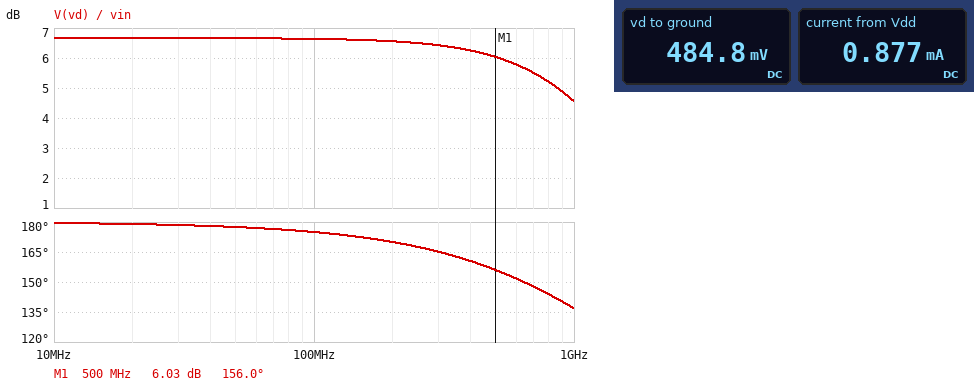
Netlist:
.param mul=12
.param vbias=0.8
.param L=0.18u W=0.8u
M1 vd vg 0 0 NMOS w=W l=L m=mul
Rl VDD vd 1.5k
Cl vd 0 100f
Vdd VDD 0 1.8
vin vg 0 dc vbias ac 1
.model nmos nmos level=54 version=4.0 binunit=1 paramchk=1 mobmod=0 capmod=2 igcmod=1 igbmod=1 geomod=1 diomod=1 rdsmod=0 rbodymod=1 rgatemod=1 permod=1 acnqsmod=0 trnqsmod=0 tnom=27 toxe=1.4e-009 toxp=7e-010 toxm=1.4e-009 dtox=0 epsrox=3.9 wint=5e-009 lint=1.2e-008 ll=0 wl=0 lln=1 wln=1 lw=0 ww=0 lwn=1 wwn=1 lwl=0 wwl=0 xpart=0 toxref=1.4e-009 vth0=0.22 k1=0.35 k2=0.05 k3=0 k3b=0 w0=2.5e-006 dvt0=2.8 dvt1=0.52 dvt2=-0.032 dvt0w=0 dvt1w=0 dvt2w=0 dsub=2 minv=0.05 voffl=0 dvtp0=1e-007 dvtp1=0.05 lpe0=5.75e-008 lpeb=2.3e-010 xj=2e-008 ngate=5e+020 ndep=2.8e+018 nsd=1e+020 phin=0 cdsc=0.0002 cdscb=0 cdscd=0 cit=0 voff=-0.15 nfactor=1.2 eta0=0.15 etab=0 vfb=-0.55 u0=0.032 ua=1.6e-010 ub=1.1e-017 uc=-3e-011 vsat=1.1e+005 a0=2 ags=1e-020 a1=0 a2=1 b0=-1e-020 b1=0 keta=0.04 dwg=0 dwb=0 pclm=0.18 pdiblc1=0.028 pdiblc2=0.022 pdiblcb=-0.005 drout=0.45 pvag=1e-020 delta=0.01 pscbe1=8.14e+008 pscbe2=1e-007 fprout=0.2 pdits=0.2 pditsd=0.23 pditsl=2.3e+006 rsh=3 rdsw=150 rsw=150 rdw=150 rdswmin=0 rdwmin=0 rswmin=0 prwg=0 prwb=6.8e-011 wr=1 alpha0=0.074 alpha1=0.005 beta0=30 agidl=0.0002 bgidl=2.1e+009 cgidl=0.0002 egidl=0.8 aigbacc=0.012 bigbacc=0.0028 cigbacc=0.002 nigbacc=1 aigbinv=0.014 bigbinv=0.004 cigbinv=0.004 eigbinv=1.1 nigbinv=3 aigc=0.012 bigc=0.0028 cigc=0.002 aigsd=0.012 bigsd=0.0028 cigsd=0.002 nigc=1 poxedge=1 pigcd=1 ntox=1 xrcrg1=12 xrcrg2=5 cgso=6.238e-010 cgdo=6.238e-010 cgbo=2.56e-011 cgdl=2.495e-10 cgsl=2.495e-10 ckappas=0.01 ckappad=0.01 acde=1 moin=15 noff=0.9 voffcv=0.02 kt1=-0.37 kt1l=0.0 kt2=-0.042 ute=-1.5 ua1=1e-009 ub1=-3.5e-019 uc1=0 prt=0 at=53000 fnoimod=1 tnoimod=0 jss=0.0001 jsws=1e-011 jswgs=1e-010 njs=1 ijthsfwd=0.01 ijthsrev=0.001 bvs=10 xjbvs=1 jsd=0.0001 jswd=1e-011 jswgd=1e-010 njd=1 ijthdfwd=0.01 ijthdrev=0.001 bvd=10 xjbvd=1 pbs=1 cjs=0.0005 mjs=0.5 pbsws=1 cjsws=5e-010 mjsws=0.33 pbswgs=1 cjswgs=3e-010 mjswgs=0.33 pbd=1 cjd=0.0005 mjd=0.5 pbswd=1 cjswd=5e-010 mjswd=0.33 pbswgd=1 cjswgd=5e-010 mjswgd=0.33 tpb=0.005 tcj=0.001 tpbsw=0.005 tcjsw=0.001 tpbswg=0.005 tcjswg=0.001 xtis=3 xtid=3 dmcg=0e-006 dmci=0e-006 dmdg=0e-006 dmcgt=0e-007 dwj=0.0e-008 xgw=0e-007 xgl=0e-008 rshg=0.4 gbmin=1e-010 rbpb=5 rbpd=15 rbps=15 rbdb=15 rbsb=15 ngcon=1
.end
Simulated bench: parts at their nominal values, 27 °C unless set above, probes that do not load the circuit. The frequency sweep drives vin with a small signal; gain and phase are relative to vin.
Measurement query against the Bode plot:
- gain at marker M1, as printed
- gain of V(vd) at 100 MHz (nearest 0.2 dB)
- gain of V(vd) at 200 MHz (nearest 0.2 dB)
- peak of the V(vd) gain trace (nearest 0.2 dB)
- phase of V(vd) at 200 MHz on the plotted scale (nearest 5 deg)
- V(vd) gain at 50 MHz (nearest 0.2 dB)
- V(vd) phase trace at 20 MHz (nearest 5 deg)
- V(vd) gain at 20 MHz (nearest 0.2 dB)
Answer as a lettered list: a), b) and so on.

a) 6.03 dB
b) 6.6 dB
c) 6.6 dB
d) 6.6 dB
e) 170 deg
f) 6.6 dB
g) 180 deg
h) 6.6 dB
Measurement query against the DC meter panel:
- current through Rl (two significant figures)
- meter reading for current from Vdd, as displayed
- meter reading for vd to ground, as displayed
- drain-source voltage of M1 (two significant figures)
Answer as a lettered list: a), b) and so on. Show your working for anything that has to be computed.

a) (1.8 V - 484.8 mV) / 1.5 kΩ = 880 µA
b) 0.877 mA
c) 484.8 mV
d) 484.8 mV = 480 mV
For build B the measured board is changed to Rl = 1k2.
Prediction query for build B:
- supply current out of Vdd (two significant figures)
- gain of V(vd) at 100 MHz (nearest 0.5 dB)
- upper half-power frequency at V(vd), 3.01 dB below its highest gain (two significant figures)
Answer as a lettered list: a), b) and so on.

a) 920 µA
b) 6.0 dB
c) 1.4 GHz
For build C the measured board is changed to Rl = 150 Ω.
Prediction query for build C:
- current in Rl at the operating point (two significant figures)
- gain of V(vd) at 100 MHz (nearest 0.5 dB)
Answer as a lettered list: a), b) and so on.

a) 1.1 mA
b) -9.5 dB
